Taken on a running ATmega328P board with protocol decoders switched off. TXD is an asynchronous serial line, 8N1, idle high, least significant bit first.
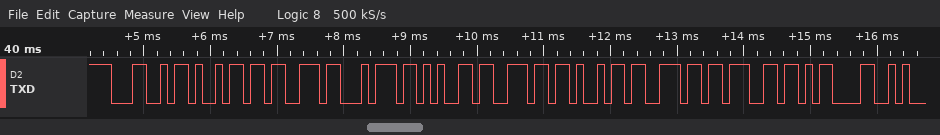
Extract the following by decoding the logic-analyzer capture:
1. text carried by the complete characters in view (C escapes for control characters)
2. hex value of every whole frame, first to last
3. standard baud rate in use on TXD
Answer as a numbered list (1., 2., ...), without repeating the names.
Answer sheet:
1. "Listening\r"
2. 4C 69 73 74 65 6E 69 6E 67 0D
3. 9600 baud
